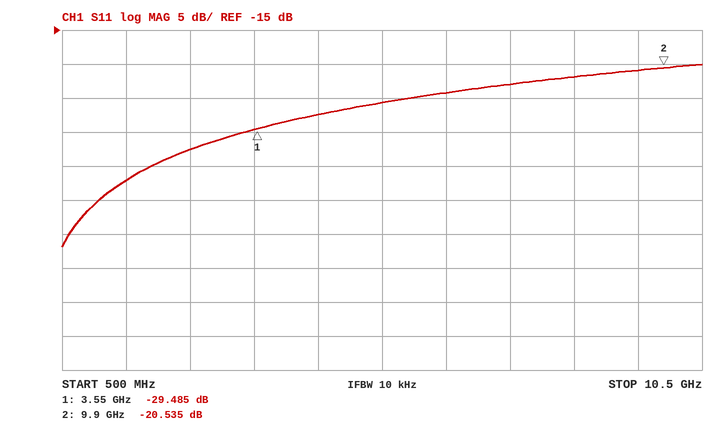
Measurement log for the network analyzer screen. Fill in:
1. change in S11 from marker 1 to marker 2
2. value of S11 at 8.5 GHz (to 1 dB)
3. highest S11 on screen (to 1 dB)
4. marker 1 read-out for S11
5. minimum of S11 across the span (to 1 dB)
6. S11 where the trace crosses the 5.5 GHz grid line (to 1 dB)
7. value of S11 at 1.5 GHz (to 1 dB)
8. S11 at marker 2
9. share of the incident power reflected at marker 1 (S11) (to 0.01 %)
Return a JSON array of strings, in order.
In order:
["8.950 dB", "-22 dB", "-20 dB", "-29.485 dB", "-47 dB", "-26 dB", "-37 dB", "-20.535 dB", "0.11 %"]
